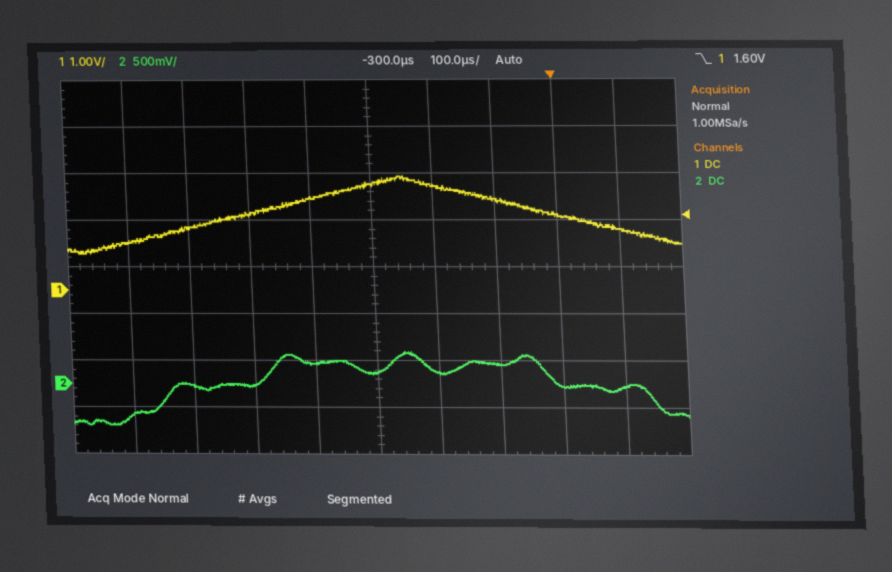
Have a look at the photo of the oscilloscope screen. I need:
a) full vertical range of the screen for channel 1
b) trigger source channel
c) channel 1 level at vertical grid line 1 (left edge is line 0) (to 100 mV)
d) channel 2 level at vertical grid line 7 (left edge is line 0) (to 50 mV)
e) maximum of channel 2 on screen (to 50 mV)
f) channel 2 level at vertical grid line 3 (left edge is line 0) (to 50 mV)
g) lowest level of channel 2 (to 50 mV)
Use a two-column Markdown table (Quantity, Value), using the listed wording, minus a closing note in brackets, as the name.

| Quantity | Value |
|---|---|
| full vertical range of the screen for channel 1 | 8 V |
| trigger source channel | channel 1 |
| channel 1 level at vertical grid line 1 (left edge is line 0) | 1.0 V |
| channel 2 level at vertical grid line 7 (left edge is line 0) | 200 mV |
| maximum of channel 2 on screen | 350 mV |
| channel 2 level at vertical grid line 3 (left edge is line 0) | 0 mV |
| lowest level of channel 2 | -450 mV |
